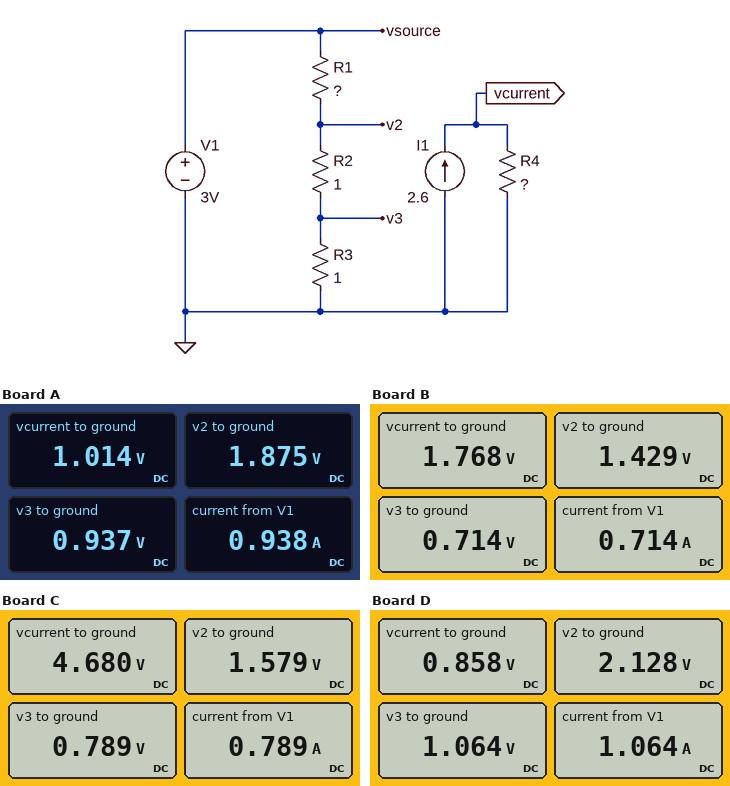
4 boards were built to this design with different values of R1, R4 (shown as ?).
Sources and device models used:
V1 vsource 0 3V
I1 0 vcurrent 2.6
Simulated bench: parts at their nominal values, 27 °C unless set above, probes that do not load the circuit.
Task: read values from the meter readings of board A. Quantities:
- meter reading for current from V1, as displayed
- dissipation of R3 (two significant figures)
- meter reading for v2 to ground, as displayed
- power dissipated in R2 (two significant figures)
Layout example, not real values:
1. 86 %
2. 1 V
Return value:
1. 0.938 A
2. 880 mW
3. 1.875 V
4. 880 mW
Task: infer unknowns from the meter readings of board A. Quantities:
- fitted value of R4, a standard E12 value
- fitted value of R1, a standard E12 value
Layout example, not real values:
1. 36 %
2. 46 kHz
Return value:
1. 0.39 Ω
2. 1.2 Ω
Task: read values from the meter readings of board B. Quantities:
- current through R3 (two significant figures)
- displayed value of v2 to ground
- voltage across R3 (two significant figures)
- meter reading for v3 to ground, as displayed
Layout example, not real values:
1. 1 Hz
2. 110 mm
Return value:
1. 710 mA
2. 1.429 V
3. 710 mV
4. 0.714 V
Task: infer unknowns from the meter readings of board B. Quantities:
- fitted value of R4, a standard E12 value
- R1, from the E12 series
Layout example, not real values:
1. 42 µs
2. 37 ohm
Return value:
1. 0.68 Ω
2. 2.2 Ω
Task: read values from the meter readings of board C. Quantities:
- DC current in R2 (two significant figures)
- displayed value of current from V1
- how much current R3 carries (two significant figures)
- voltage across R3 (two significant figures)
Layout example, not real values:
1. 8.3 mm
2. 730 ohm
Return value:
1. 790 mA
2. 0.789 A
3. 790 mA
4. 790 mV
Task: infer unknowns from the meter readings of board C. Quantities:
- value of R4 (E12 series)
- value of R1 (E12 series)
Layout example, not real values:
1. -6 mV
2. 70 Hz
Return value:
1. 1.8 Ω
2. 1.8 Ω
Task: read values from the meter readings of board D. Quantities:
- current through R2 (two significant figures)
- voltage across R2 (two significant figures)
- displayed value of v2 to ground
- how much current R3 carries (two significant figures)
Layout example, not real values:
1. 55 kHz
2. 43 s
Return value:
1. 1.1 A
2. 1.1 V
3. 2.128 V
4. 1.1 A
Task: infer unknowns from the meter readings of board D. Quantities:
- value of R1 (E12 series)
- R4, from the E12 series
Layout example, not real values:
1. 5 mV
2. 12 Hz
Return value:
1. 0.82 Ω
2. 0.33 Ω
